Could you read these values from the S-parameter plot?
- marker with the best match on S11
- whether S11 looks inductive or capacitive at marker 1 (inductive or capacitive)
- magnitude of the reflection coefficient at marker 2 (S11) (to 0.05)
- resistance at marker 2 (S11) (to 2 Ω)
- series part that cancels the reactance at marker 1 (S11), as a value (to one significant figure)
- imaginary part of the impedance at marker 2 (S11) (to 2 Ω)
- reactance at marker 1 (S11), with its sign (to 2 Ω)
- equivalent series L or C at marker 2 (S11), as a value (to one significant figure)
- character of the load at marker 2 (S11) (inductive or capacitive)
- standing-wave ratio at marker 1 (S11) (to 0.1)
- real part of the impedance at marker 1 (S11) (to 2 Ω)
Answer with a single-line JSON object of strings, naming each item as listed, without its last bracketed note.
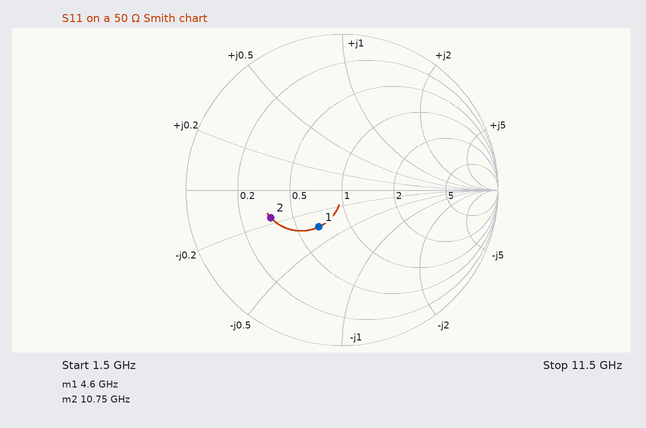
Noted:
{"marker with the best match on S11": "marker 1", "whether S11 looks inductive or capacitive at marker 1": "capacitive", "magnitude of the reflection coefficient at marker 2 (S11)": "0.50", "resistance at marker 2 (S11)": "18 Ω", "series part that cancels the reactance at marker 1 (S11), as a value": "600 pH", "imaginary part of the impedance at marker 2 (S11)": "-8 Ω", "reactance at marker 1 (S11), with its sign": "-18 Ω", "equivalent series L or C at marker 2 (S11), as a value": "2 pF", "character of the load at marker 2 (S11)": "capacitive", "standing-wave ratio at marker 1 (S11)": "1.8", "real part of the impedance at marker 1 (S11)": "34 Ω"}
